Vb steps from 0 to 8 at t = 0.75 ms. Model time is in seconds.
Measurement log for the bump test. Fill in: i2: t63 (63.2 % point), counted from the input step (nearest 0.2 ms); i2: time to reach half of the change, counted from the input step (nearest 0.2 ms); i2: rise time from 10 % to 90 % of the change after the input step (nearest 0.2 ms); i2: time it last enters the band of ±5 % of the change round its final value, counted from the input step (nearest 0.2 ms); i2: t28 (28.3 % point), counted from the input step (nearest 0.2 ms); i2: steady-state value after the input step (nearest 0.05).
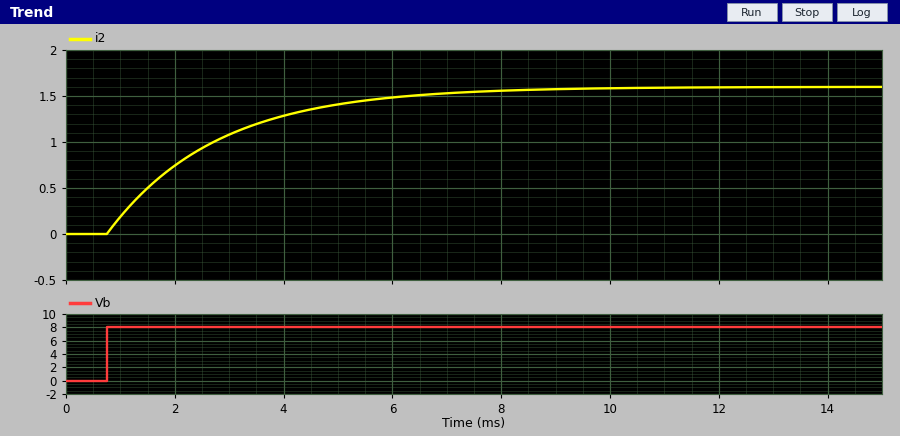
2.0 ms
1.4 ms
4.4 ms
6.0 ms
0.6 ms
1.60
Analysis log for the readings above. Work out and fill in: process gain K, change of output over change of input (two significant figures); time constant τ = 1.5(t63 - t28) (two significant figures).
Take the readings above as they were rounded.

0.20
2.1 ms
